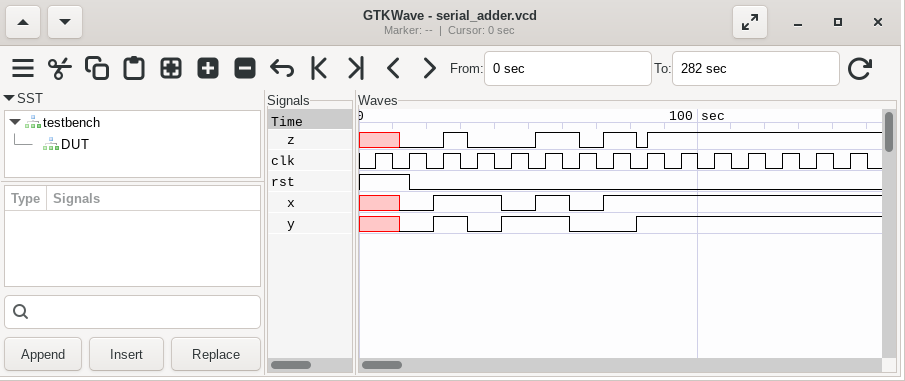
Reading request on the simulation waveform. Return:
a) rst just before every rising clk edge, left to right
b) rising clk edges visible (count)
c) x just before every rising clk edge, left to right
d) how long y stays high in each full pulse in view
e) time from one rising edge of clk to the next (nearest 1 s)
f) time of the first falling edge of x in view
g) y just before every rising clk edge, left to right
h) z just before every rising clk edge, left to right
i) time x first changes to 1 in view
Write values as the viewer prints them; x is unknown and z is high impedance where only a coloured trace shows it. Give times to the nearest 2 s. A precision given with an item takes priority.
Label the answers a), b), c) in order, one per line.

a) 1 1 0 0 0 0 0 0 0 0 0 0 0 0 0
b) 15
c) x 0 1 1 0 1 0 1 1 1 1 1 1 1 1
d) 10 s, 20 s
e) 10 s
f) 42 s
g) x 0 1 0 1 1 0 0 1 1 1 1 1 1 1
h) x 0 0 0 0 1 1 1 0 1 1 1 1 1 1
i) 22 s
